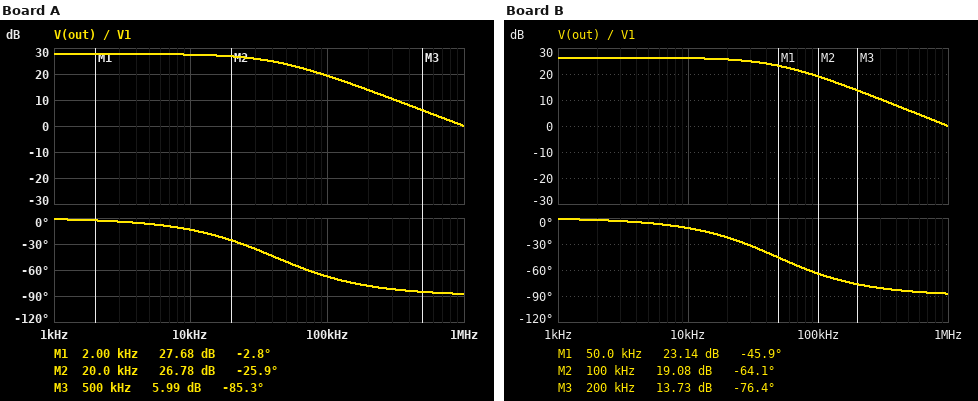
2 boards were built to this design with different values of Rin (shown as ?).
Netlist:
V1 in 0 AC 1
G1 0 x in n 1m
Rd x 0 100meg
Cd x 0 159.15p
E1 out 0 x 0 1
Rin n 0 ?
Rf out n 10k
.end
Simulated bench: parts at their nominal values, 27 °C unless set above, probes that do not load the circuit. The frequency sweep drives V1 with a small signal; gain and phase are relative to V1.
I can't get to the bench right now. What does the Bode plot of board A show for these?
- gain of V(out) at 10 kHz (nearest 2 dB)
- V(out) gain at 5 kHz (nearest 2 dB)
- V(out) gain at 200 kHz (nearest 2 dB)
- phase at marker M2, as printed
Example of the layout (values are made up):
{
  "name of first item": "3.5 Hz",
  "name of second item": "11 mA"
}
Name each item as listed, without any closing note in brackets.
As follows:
{
  "gain of V(out) at 10 kHz": "28 dB",
  "V(out) gain at 5 kHz": "28 dB",
  "V(out) gain at 200 kHz": "14 dB",
  "phase at marker M2, as printed": "-25.9 deg"
}
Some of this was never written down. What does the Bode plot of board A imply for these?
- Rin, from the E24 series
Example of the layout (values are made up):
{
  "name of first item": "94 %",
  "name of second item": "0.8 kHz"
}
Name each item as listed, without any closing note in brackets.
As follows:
{
  "Rin, from the E24 series": "430 Ω"
}
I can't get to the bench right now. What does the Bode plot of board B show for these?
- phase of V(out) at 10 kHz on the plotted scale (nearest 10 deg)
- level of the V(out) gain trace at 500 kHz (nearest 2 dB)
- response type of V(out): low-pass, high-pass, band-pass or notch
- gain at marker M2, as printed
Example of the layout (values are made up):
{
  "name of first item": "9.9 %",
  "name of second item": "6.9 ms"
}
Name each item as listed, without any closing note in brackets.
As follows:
{
  "phase of V(out) at 10 kHz on the plotted scale": "-10 deg",
  "level of the V(out) gain trace at 500 kHz": "6 dB",
  "response type of V(out): low-pass, high-pass, band-pass or notch": "low-pass",
  "gain at marker M2, as printed": "19.08 dB"
}
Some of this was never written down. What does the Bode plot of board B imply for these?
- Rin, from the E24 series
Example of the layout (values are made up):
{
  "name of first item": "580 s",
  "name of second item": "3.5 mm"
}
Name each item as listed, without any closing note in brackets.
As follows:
{
  "Rin, from the E24 series": "510 Ω"
}
